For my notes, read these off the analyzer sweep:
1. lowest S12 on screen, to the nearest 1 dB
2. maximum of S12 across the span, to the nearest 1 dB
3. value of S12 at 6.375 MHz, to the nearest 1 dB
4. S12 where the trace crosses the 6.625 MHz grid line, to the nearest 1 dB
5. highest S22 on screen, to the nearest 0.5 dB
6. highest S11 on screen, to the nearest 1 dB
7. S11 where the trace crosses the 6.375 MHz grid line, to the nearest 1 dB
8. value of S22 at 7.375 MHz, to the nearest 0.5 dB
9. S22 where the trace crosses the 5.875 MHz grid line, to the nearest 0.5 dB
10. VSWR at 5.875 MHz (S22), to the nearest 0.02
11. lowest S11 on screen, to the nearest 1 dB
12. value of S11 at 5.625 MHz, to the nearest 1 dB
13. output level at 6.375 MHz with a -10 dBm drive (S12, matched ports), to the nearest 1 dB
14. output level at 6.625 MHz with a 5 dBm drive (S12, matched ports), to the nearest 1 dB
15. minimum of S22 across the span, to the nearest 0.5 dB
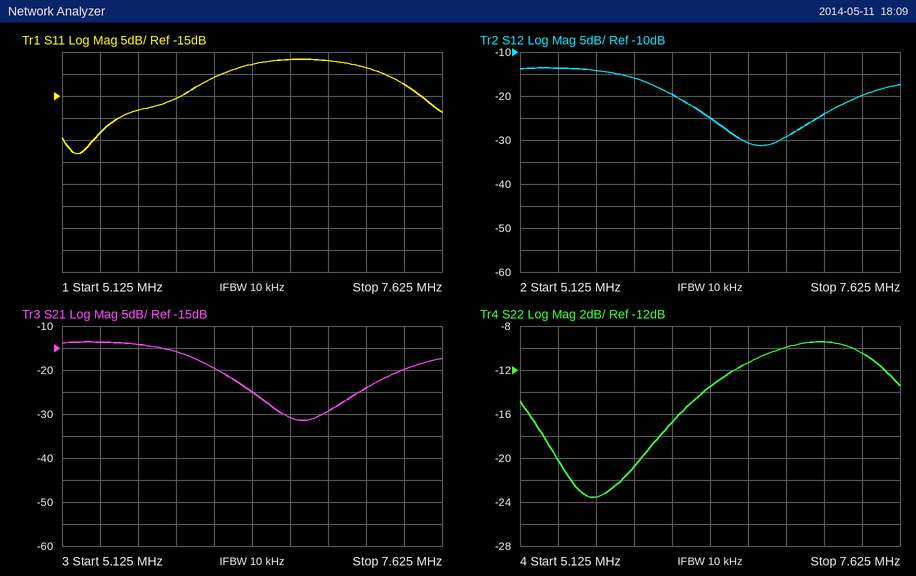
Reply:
-31 dB
-14 dB
-25 dB
-31 dB
-9.5 dB
-7 dB
-8 dB
-10.5 dB
-21.0 dB
1.20
-28 dB
-18 dB
-35 dBm
-26 dBm
-23.5 dB
